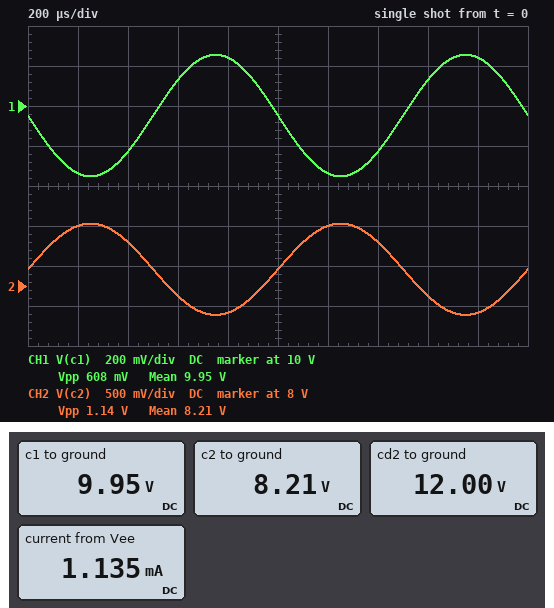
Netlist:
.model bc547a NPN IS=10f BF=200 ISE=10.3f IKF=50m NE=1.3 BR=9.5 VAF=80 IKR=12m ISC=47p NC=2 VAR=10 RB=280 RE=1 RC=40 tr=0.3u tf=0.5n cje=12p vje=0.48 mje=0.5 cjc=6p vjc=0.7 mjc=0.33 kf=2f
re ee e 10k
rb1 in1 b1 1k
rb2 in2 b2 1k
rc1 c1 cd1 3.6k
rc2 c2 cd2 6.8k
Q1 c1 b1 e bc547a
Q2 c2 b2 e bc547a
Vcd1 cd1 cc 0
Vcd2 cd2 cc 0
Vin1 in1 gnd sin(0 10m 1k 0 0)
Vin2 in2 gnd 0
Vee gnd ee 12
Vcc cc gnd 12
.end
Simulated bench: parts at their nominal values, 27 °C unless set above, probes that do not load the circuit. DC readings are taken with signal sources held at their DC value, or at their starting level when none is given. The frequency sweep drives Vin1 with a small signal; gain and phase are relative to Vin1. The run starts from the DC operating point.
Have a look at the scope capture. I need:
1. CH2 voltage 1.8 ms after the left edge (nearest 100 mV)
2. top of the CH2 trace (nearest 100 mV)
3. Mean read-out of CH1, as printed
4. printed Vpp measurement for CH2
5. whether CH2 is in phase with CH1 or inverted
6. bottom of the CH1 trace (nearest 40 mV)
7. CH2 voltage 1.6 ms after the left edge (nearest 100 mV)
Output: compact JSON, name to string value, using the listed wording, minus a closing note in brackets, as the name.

{"CH2 voltage 1.8 ms after the left edge": "7.7 V", "top of the CH2 trace": "8.8 V", "Mean read-out of CH1, as printed": "9.95 V", "printed Vpp measurement for CH2": "1.14 V", "whether CH2 is in phase with CH1 or inverted": "inverted", "bottom of the CH1 trace": "9.64 V", "CH2 voltage 1.6 ms after the left edge": "7.9 V"}
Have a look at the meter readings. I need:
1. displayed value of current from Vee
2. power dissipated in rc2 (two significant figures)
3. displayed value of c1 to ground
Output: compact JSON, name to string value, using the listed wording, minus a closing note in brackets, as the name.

{"displayed value of current from Vee": "1.135 mA", "power dissipated in rc2": "2.1 mW", "displayed value of c1 to ground": "9.95 V"}
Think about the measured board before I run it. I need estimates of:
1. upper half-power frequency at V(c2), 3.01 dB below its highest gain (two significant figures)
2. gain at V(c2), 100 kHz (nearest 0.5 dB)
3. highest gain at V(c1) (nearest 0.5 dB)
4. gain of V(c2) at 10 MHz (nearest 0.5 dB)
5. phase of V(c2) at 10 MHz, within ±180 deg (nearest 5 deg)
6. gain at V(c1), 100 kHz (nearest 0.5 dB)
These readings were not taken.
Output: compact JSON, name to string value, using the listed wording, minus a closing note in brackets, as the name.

{"upper half-power frequency at V(c2), 3.01 dB below its highest gain": "460 kHz", "gain at V(c2), 100 kHz": "35.0 dB", "highest gain at V(c1)": "29.5 dB", "gain of V(c2) at 10 MHz": "6.5 dB", "phase of V(c2) at 10 MHz, within ±180 deg": "-95 deg", "gain at V(c1), 100 kHz": "29.5 dB"}
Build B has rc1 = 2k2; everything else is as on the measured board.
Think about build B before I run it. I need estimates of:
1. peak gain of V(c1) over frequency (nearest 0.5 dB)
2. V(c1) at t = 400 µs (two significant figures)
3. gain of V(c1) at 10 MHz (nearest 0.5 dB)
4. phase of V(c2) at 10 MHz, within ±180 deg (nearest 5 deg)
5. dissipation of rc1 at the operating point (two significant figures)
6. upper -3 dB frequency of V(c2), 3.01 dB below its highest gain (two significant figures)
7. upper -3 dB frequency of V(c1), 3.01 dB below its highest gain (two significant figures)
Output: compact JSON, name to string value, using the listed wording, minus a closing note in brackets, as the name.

{"peak gain of V(c1) over frequency": "25.5 dB", "V(c1) at t = 400 µs": "11 V", "gain of V(c1) at 10 MHz": "3.5 dB", "phase of V(c2) at 10 MHz, within ±180 deg": "-100 deg", "dissipation of rc1 at the operating point": "720 µW", "upper -3 dB frequency of V(c2), 3.01 dB below its highest gain": "510 kHz", "upper -3 dB frequency of V(c1), 3.01 dB below its highest gain": "520 kHz"}
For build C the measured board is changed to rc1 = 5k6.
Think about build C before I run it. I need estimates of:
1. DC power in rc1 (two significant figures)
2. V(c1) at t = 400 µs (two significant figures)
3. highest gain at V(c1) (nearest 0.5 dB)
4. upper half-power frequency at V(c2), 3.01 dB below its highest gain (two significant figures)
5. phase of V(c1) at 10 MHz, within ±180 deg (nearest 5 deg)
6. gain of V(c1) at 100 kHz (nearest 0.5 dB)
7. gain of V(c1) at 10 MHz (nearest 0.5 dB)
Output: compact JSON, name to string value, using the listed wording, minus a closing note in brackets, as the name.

{"DC power in rc1": "1.8 mW", "V(c1) at t = 400 µs": "8.6 V", "highest gain at V(c1)": "33.5 dB", "upper half-power frequency at V(c2), 3.01 dB below its highest gain": "390 kHz", "phase of V(c1) at 10 MHz, within ±180 deg": "85 deg", "gain of V(c1) at 100 kHz": "33.0 dB", "gain of V(c1) at 10 MHz": "7.0 dB"}
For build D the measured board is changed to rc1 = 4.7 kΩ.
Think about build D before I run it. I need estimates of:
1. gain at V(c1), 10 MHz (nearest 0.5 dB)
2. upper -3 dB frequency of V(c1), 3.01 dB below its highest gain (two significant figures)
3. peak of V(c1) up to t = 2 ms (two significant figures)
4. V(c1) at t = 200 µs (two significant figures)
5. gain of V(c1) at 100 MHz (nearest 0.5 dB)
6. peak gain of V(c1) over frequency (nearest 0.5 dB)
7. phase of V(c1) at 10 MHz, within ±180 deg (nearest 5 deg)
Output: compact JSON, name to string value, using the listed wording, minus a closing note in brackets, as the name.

{"gain at V(c1), 10 MHz": "6.5 dB", "upper -3 dB frequency of V(c1), 3.01 dB below its highest gain": "420 kHz", "peak of V(c1) up to t = 2 ms": "9.7 V", "V(c1) at t = 200 µs": "9.0 V", "gain of V(c1) at 100 MHz": "-6.0 dB", "peak gain of V(c1) over frequency": "32.0 dB", "phase of V(c1) at 10 MHz, within ±180 deg": "85 deg"}
